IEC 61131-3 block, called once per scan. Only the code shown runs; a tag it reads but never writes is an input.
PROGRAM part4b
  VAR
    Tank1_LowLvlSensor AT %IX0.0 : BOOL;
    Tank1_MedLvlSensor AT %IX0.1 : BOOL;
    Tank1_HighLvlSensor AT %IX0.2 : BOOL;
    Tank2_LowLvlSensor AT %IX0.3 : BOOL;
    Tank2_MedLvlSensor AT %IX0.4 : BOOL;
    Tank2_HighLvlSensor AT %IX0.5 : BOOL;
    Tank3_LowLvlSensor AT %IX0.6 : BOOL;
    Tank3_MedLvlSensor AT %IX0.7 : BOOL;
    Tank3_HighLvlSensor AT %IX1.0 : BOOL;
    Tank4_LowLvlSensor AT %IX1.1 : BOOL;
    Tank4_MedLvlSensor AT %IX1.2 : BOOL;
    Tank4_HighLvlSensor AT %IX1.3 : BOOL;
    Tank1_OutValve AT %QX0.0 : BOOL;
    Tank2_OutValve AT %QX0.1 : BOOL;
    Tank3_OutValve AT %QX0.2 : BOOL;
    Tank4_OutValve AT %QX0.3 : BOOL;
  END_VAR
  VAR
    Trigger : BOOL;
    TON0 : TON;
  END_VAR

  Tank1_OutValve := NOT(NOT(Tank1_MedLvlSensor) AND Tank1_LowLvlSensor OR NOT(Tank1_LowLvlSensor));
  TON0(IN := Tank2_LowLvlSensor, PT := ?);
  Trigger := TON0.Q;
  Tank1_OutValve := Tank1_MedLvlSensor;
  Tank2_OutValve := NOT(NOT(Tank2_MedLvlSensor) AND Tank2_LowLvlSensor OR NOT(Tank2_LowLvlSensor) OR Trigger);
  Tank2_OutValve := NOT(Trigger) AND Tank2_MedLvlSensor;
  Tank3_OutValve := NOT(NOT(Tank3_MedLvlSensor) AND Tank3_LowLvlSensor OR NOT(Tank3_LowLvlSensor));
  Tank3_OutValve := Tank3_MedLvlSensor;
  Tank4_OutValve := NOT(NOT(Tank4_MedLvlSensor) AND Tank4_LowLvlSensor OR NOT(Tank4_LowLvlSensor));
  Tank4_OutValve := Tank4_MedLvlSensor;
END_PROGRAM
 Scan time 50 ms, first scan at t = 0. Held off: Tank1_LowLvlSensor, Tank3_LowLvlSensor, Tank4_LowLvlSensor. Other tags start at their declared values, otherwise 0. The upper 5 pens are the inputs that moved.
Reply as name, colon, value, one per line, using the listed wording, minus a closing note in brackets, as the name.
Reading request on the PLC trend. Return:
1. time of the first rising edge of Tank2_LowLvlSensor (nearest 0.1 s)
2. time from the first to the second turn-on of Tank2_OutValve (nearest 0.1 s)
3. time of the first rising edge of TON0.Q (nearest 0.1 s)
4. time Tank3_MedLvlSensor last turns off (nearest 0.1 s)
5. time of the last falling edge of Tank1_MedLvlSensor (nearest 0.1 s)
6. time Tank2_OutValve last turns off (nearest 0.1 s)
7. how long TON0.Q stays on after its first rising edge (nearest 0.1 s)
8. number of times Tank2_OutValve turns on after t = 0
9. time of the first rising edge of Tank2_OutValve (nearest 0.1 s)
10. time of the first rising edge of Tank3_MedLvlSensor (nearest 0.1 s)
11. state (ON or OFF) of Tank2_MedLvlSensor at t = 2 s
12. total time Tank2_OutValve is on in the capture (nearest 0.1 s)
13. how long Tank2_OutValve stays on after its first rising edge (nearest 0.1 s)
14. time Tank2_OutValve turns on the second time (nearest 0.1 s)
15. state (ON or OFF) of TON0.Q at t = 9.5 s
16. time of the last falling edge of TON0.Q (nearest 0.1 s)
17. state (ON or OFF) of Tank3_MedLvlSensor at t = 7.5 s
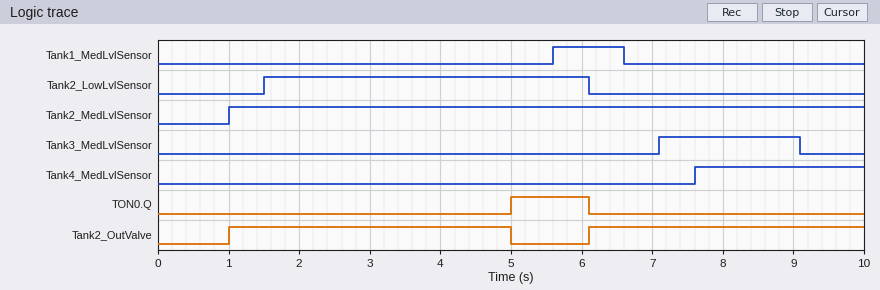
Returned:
time of the first rising edge of Tank2_LowLvlSensor: 1.5 s
time from the first to the second turn-on of Tank2_OutValve: 5.1 s
time of the first rising edge of TON0.Q: 5.0 s
time Tank3_MedLvlSensor last turns off: 9.1 s
time of the last falling edge of Tank1_MedLvlSensor: 6.6 s
time Tank2_OutValve last turns off: 5.0 s
how long TON0.Q stays on after its first rising edge: 1.1 s
number of times Tank2_OutValve turns on after t = 0: 2
time of the first rising edge of Tank2_OutValve: 1.0 s
time of the first rising edge of Tank3_MedLvlSensor: 7.1 s
state (ON or OFF) of Tank2_MedLvlSensor at t = 2 s: ON
total time Tank2_OutValve is on in the capture: 7.9 s
how long Tank2_OutValve stays on after its first rising edge: 4.0 s
time Tank2_OutValve turns on the second time: 6.1 s
state (ON or OFF) of TON0.Q at t = 9.5 s: OFF
time of the last falling edge of TON0.Q: 6.1 s
state (ON or OFF) of Tank3_MedLvlSensor at t = 7.5 s: ON
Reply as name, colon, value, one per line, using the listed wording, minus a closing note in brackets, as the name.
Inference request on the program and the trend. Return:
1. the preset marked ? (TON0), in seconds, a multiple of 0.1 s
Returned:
the preset marked ? (TON0), in seconds, a multiple of 0.1 s: 3.5 s
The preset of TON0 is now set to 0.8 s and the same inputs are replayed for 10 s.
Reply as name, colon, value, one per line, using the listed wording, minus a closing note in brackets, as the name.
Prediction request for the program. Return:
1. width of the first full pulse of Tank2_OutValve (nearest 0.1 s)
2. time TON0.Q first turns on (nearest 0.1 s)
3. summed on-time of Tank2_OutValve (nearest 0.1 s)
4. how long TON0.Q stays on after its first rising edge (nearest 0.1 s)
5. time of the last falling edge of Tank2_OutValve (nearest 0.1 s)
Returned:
width of the first full pulse of Tank2_OutValve: 1.3 s
time TON0.Q first turns on: 2.3 s
summed on-time of Tank2_OutValve: 5.2 s
how long TON0.Q stays on after its first rising edge: 3.8 s
time of the last falling edge of Tank2_OutValve: 2.3 s
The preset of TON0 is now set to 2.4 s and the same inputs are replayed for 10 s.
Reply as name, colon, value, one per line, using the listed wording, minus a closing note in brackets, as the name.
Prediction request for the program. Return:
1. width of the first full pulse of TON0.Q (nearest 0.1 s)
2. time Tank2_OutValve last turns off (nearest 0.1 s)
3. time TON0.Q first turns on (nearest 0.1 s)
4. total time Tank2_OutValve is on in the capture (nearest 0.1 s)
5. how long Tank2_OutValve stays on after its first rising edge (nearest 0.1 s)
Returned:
width of the first full pulse of TON0.Q: 2.2 s
time Tank2_OutValve last turns off: 3.9 s
time TON0.Q first turns on: 3.9 s
total time Tank2_OutValve is on in the capture: 6.8 s
how long Tank2_OutValve stays on after its first rising edge: 2.9 s
